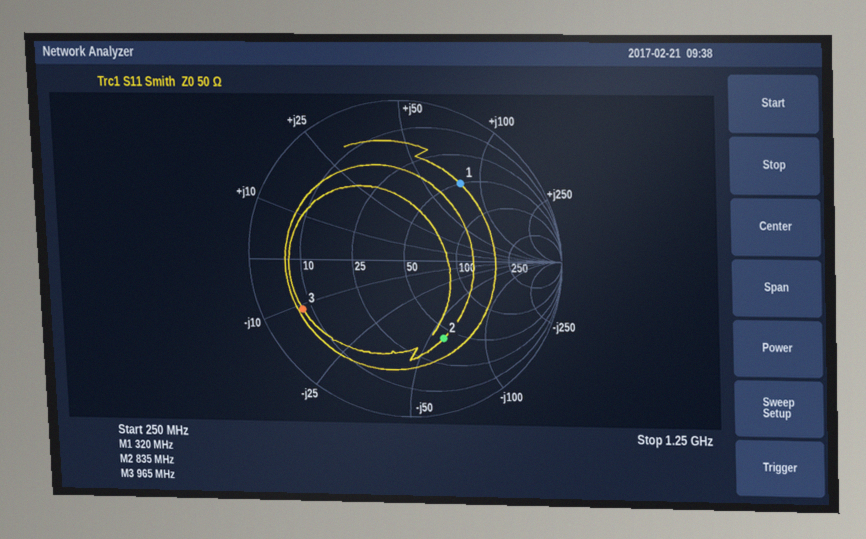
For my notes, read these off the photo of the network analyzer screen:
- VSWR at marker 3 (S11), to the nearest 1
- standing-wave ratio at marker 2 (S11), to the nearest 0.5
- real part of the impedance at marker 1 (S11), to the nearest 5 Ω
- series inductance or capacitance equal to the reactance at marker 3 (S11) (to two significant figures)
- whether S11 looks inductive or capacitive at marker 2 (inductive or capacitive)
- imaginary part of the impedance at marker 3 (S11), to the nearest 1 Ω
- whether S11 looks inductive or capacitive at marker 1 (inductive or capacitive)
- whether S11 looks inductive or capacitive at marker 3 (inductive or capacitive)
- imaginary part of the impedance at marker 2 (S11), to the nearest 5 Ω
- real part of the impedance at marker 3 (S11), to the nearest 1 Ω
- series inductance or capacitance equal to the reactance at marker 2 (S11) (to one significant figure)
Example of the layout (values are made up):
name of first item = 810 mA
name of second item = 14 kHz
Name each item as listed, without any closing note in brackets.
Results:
VSWR at marker 3 (S11), to the nearest 1 = 7
standing-wave ratio at marker 2 (S11), to the nearest 0.5 = 3.5
real part of the impedance at marker 1 (S11), to the nearest 5 Ω = 50 Ω
series inductance or capacitance equal to the reactance at marker 3 (S11) = 15 pF
whether S11 looks inductive or capacitive at marker 2 = capacitive
imaginary part of the impedance at marker 3 (S11), to the nearest 1 Ω = -11 Ω
whether S11 looks inductive or capacitive at marker 1 = inductive
whether S11 looks inductive or capacitive at marker 3 = capacitive
imaginary part of the impedance at marker 2 (S11), to the nearest 5 Ω = -60 Ω
real part of the impedance at marker 3 (S11), to the nearest 1 Ω = 8 Ω
series inductance or capacitance equal to the reactance at marker 2 (S11) = 3 pF
